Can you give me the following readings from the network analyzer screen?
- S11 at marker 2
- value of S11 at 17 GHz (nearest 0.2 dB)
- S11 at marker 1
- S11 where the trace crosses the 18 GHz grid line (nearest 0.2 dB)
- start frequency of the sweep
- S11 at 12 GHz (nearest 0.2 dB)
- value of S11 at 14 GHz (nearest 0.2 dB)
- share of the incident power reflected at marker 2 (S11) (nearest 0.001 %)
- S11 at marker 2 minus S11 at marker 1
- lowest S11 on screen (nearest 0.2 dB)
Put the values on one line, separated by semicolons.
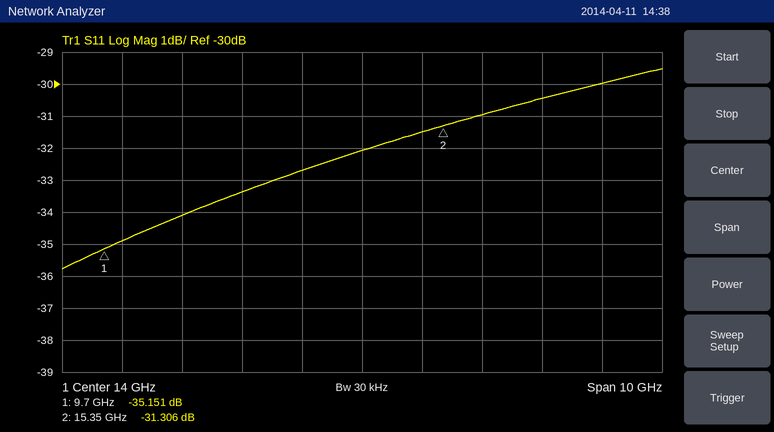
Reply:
-31.306 dB; -30.4 dB; -35.151 dB; -30.0 dB; 9 GHz; -33.4 dB; -32.0 dB; 0.074 %; 3.845 dB; -35.8 dB
